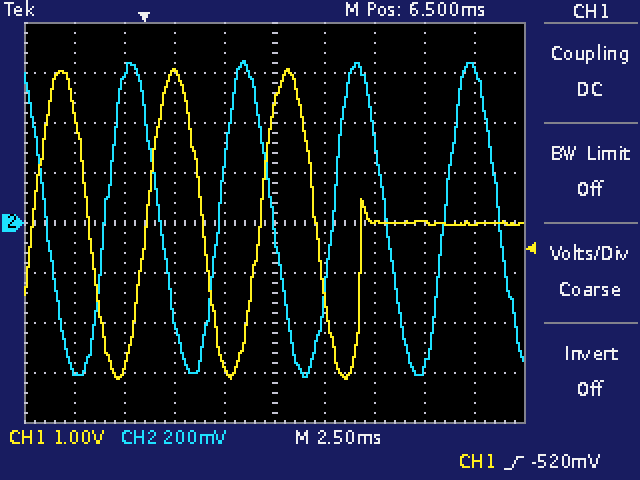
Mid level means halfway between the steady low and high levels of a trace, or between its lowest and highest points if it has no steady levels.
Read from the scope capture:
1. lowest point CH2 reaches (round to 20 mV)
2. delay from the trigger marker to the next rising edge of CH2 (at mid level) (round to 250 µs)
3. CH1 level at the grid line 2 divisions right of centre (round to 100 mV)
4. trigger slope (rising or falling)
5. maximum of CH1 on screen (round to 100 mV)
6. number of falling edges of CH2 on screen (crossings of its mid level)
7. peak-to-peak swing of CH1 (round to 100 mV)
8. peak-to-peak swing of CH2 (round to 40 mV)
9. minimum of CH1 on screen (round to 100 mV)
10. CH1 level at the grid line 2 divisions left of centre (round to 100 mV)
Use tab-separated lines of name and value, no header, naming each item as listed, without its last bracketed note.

lowest point CH2 reaches	-620 mV
delay from the trigger marker to the next rising edge of CH2 (at mid level)	3.75 ms
CH1 level at the grid line 2 divisions right of centre	0.0 V
trigger slope	rising
maximum of CH1 on screen	3.1 V
number of falling edges of CH2 on screen	5
peak-to-peak swing of CH1	6.2 V
peak-to-peak swing of CH2	1.28 V
minimum of CH1 on screen	-3.1 V
CH1 level at the grid line 2 divisions left of centre	3.0 V
